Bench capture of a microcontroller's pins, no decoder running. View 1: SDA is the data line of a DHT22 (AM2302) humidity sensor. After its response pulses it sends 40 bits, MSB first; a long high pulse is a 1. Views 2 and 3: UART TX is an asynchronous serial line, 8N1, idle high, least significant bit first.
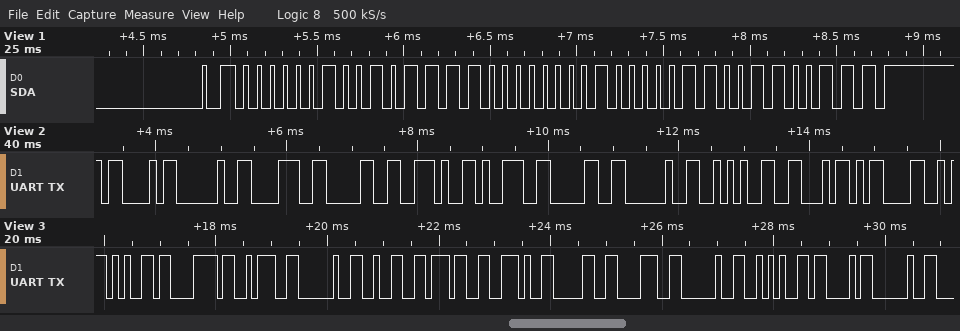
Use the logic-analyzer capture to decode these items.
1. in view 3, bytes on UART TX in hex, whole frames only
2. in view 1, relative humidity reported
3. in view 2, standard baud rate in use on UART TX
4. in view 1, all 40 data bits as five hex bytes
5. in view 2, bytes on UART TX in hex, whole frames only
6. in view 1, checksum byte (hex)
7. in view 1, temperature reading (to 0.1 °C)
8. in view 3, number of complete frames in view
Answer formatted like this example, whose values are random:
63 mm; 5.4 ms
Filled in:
65 78 3A 20 32 37 2E 30 38 20 2A 43 20; 60.6 %; 9600 baud; 02 5E 01 06 67; 0x43 0x20 0x38 0x30 0x2E 0x39 0x30 0x20 0x2A 0x46 0x0D; 0x67; 26.2 °C; 13
